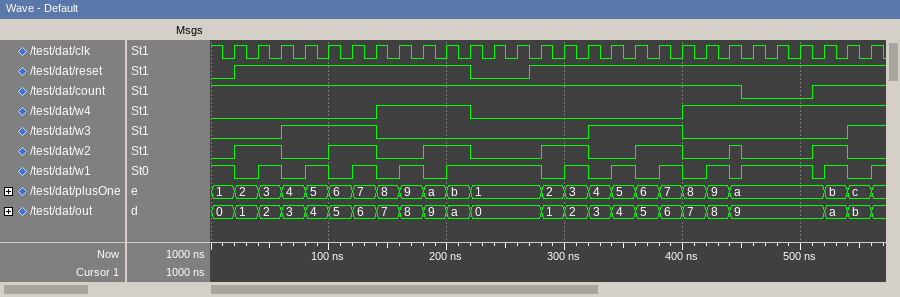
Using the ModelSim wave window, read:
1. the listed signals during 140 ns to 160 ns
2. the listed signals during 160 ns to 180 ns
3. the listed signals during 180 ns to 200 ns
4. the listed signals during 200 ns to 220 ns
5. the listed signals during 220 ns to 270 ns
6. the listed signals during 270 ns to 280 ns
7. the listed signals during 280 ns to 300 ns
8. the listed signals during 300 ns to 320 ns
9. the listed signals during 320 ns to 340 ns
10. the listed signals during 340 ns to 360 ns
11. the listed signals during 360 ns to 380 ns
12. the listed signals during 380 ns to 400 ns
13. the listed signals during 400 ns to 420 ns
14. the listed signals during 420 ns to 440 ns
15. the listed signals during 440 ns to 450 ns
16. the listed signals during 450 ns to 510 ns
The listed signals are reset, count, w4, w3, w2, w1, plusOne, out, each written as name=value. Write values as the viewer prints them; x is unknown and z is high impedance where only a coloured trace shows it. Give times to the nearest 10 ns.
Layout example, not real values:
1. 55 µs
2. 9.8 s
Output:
1. reset=1, count=1, w4=1, w3=0, w2=0, w1=0, plusOne=8, out=7
2. reset=1, count=1, w4=1, w3=0, w2=0, w1=1, plusOne=9, out=8
3. reset=1, count=1, w4=1, w3=0, w2=1, w1=0, plusOne=a, out=9
4. reset=1, count=1, w4=1, w3=0, w2=1, w1=1, plusOne=b, out=a
5. reset=0, count=1, w4=0, w3=0, w2=0, w1=1, plusOne=1, out=0
6. reset=1, count=1, w4=0, w3=0, w2=0, w1=1, plusOne=1, out=0
7. reset=1, count=1, w4=0, w3=0, w2=1, w1=0, plusOne=2, out=1
8. reset=1, count=1, w4=0, w3=0, w2=1, w1=1, plusOne=3, out=2
9. reset=1, count=1, w4=0, w3=1, w2=0, w1=0, plusOne=4, out=3
10. reset=1, count=1, w4=0, w3=1, w2=0, w1=1, plusOne=5, out=4
11. reset=1, count=1, w4=0, w3=1, w2=1, w1=0, plusOne=6, out=5
12. reset=1, count=1, w4=0, w3=1, w2=1, w1=1, plusOne=7, out=6
13. reset=1, count=1, w4=1, w3=0, w2=0, w1=0, plusOne=8, out=7
14. reset=1, count=1, w4=1, w3=0, w2=0, w1=1, plusOne=9, out=8
15. reset=1, count=1, w4=1, w3=0, w2=1, w1=0, plusOne=a, out=9
16. reset=1, count=0, w4=1, w3=0, w2=0, w1=1, plusOne=a, out=9
